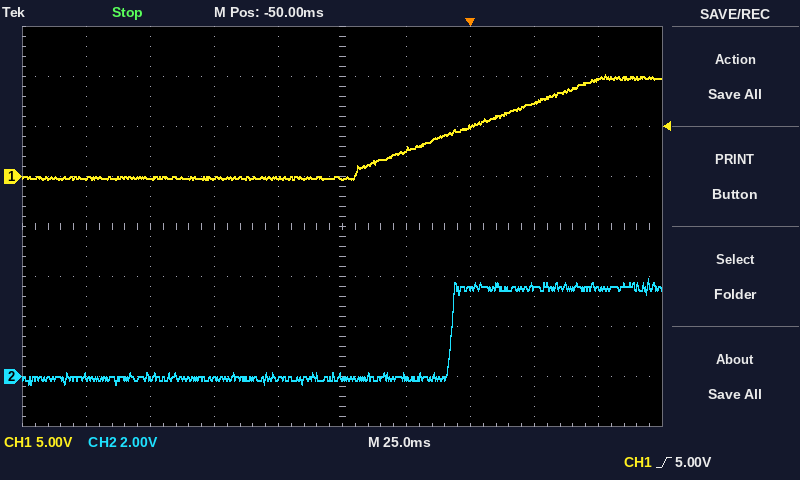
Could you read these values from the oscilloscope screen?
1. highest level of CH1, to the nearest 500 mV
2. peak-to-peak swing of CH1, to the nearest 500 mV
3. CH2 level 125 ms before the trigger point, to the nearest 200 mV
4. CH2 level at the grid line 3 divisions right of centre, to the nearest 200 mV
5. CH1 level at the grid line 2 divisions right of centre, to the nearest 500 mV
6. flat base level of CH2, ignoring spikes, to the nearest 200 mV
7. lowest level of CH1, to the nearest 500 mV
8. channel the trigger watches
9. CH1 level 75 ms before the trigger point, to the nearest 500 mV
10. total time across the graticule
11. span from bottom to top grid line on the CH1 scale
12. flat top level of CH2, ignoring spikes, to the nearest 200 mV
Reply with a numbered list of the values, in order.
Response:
1. 10.0 V
2. 10.5 V
3. 0.0 V
4. 3.6 V
5. 5.0 V
6. 0.0 V
7. -500 mV
8. CH1
9. 0.0 V
10. 250 ms
11. 40 V
12. 3.6 V
